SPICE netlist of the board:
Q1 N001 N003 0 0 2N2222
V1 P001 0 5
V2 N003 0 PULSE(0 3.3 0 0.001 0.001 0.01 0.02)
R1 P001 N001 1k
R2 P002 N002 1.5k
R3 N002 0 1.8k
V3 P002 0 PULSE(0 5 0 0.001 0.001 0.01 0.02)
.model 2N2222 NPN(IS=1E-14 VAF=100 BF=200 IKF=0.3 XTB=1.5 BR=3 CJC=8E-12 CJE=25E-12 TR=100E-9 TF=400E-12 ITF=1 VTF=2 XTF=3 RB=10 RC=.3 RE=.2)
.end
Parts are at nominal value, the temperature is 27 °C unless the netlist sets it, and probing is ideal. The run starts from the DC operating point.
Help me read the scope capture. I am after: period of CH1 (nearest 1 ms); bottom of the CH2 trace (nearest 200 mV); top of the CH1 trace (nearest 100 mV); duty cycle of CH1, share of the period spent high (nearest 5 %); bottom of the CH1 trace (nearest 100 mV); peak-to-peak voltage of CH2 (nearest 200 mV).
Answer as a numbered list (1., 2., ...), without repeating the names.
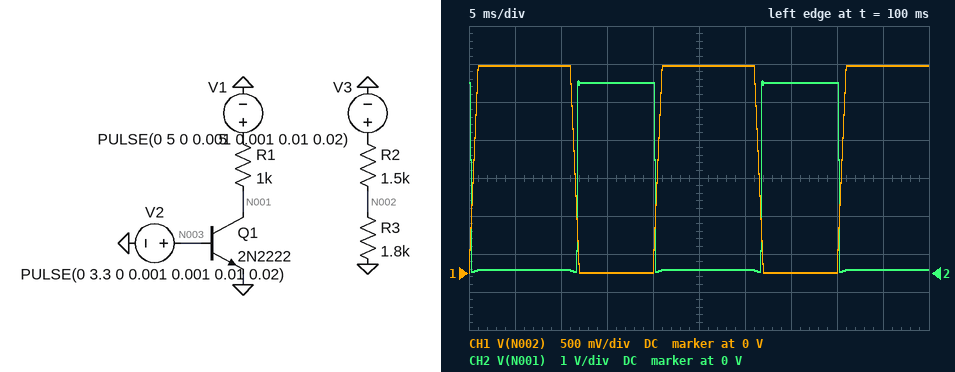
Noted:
1. 20 ms
2. 0 V
3. 2.7 V
4. 55 %
5. 0 V
6. 5.0 V
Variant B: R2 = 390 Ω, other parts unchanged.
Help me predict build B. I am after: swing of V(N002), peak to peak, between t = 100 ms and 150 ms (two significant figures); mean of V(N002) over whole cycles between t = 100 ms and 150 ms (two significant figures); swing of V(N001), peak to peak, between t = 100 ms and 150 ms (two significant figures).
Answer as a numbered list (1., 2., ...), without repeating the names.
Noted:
1. 4.1 V
2. 2.3 V
3. 5.0 V
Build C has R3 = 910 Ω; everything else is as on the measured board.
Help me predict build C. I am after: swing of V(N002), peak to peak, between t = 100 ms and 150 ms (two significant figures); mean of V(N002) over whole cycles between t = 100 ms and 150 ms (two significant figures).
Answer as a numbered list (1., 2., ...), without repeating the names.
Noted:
1. 1.9 V
2. 1.0 V
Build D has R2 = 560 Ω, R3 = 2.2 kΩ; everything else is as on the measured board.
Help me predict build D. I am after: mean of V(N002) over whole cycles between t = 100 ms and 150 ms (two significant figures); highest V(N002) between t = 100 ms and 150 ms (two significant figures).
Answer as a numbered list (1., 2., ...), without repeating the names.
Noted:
1. 2.2 V
2. 4.0 V
